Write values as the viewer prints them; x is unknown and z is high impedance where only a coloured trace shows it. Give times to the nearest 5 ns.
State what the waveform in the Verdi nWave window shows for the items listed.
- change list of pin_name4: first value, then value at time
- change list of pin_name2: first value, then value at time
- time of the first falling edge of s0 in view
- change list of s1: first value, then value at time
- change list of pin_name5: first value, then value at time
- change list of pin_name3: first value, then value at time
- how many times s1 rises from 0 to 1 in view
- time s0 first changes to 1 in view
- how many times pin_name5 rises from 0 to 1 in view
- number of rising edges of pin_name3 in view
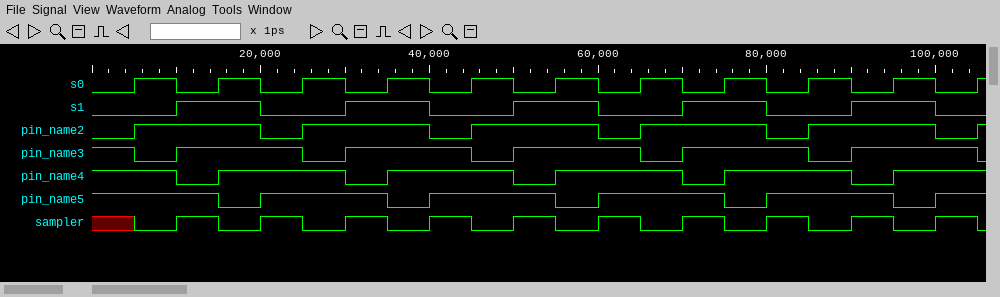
1, 0 at 10 ns, 1 at 15 ns, 0 at 30 ns, 1 at 35 ns, 0 at 50 ns, 1 at 55 ns, 0 at 70 ns, 1 at 75 ns, 0 at 90 ns, 1 at 95 ns
0, 1 at 5 ns, 0 at 20 ns, 1 at 25 ns, 0 at 40 ns, 1 at 45 ns, 0 at 60 ns, 1 at 65 ns, 0 at 80 ns, 1 at 85 ns, 0 at 100 ns, 1 at 105 ns
10 ns
0, 1 at 10 ns, 0 at 20 ns, 1 at 30 ns, 0 at 40 ns, 1 at 50 ns, 0 at 60 ns, 1 at 70 ns, 0 at 80 ns, 1 at 90 ns, 0 at 100 ns
1, 0 at 15 ns, 1 at 20 ns, 0 at 35 ns, 1 at 40 ns, 0 at 55 ns, 1 at 60 ns, 0 at 75 ns, 1 at 80 ns, 0 at 95 ns, 1 at 100 ns
1, 0 at 5 ns, 1 at 10 ns, 0 at 25 ns, 1 at 30 ns, 0 at 45 ns, 1 at 50 ns, 0 at 65 ns, 1 at 70 ns, 0 at 85 ns, 1 at 90 ns, 0 at 105 ns
5
5 ns
5
5
